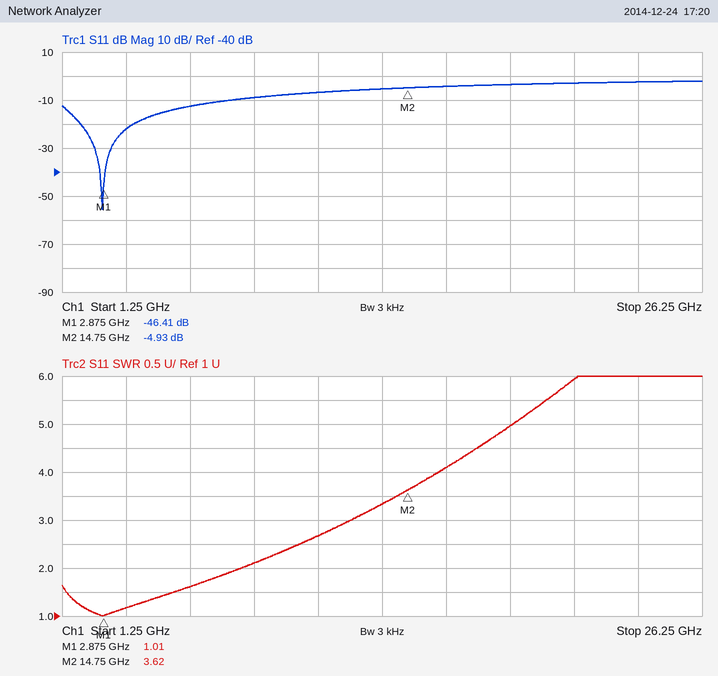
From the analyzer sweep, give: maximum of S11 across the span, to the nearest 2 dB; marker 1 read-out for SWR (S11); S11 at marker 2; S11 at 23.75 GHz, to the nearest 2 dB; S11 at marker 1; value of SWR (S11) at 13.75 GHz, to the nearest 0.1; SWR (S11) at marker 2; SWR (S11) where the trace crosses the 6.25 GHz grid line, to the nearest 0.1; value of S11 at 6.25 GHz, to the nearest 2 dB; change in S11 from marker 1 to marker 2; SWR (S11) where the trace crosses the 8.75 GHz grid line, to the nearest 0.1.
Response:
-2 dB
1.01
-4.93 dB
-2 dB
-46.41 dB
3.3
3.62
1.6
-12 dB
41.48 dB
2.1
